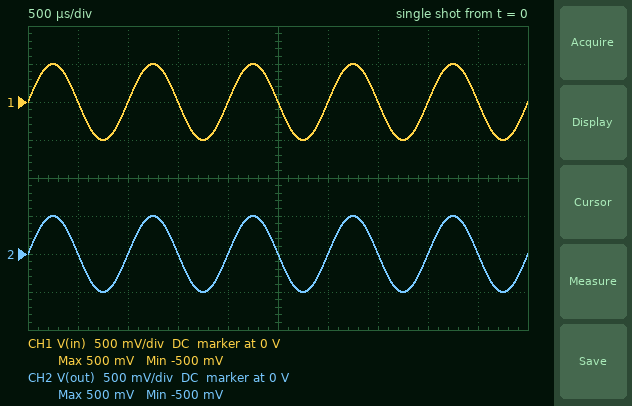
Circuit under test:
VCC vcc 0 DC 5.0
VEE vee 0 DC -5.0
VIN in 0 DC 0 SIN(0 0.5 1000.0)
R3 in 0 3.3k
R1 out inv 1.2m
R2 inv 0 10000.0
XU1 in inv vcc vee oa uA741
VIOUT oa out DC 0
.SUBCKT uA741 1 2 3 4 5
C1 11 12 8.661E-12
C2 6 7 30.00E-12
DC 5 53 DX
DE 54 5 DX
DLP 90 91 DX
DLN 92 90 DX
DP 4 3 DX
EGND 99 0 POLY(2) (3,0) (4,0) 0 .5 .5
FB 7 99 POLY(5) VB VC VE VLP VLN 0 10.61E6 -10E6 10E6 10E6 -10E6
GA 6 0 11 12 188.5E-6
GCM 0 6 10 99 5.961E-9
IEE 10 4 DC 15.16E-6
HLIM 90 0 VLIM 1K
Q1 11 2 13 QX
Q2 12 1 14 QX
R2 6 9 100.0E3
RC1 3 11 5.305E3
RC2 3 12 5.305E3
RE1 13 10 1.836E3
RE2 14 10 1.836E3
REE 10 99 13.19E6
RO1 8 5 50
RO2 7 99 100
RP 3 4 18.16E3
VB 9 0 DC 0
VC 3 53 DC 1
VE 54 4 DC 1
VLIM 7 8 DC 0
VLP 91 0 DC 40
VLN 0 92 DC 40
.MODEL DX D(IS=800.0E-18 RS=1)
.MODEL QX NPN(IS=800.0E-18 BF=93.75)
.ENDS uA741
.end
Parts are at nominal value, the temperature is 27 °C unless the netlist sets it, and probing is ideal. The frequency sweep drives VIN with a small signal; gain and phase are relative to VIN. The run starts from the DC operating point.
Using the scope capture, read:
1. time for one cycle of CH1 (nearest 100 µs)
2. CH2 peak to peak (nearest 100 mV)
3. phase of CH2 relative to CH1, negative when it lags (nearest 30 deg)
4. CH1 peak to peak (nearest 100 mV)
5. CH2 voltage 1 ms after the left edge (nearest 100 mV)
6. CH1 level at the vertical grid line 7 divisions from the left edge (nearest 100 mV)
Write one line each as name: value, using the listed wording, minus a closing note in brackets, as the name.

time for one cycle of CH1: 1.0 ms
CH2 peak to peak: 1.0 V
phase of CH2 relative to CH1, negative when it lags: 0 deg
CH1 peak to peak: 1.0 V
CH2 voltage 1 ms after the left edge: 0 V
CH1 level at the vertical grid line 7 divisions from the left edge: 0 V
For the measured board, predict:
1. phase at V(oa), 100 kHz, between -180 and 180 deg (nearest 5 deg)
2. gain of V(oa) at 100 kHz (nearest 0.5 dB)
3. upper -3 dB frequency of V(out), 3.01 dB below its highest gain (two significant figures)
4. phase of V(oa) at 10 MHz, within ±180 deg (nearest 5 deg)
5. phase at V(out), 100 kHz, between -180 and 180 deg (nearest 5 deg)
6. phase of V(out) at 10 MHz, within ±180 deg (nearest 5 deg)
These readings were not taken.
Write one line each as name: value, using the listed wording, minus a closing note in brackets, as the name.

phase at V(oa), 100 kHz, between -180 and 180 deg: -5 deg
gain of V(oa) at 100 kHz: 0 dB
upper -3 dB frequency of V(out), 3.01 dB below its highest gain: 1.4 MHz
phase of V(oa) at 10 MHz, within ±180 deg: -170 deg
phase at V(out), 100 kHz, between -180 and 180 deg: -5 deg
phase of V(out) at 10 MHz, within ±180 deg: -170 deg
